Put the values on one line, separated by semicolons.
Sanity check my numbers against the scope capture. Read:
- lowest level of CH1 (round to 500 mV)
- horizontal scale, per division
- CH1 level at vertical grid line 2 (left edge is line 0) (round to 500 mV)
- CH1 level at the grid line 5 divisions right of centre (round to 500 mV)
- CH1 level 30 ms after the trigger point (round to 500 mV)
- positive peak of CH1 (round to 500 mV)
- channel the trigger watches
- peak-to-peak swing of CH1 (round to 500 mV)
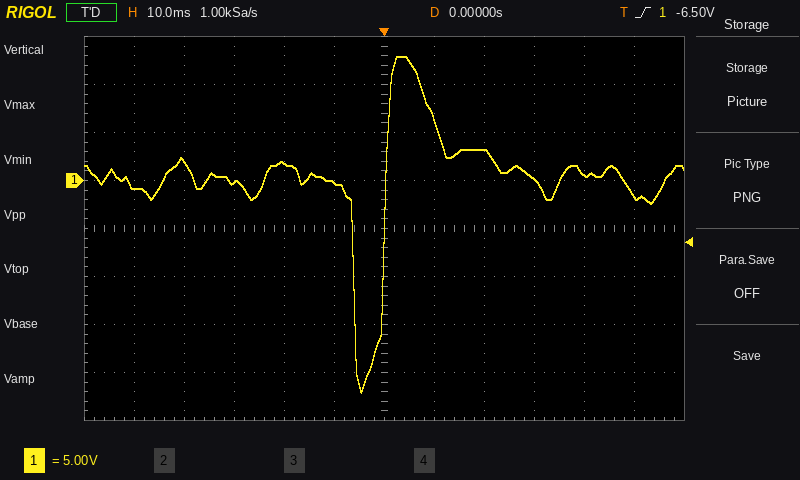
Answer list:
-22.0 V; 10 ms; 2.0 V; -1.5 V; 0.0 V; 13.0 V; CH1; 35.0 V
